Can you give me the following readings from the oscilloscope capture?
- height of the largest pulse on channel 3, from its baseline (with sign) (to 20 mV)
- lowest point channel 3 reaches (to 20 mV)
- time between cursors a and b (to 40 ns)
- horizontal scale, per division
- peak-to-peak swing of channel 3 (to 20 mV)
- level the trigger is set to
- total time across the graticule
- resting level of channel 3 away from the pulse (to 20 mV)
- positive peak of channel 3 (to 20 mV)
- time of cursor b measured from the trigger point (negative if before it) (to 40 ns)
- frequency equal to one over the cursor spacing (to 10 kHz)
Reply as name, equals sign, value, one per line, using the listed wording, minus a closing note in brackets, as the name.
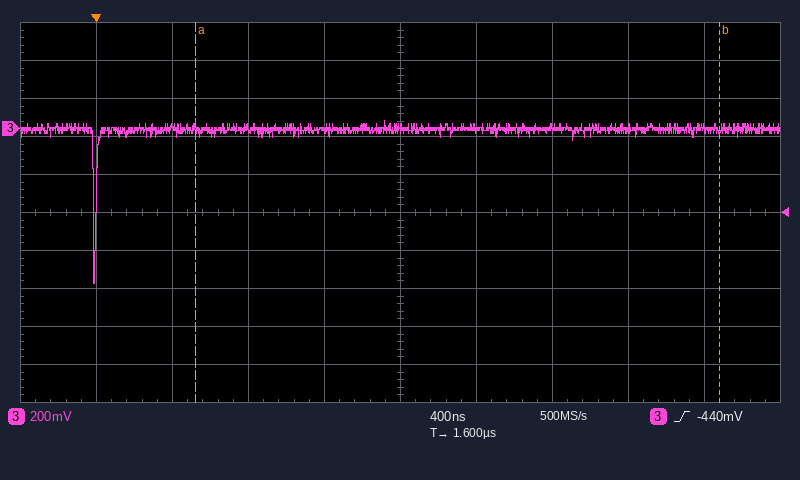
height of the largest pulse on channel 3, from its baseline (with sign) = -820 mV
lowest point channel 3 reaches = -820 mV
time between cursors a and b = 2.76 µs
horizontal scale, per division = 400 ns
peak-to-peak swing of channel 3 = 860 mV
level the trigger is set to = -440 mV
total time across the graticule = 4 µs
resting level of channel 3 away from the pulse = 0 mV
positive peak of channel 3 = 40 mV
time of cursor b measured from the trigger point (negative if before it) = +3.28 µs
frequency equal to one over the cursor spacing = 360 kHz
